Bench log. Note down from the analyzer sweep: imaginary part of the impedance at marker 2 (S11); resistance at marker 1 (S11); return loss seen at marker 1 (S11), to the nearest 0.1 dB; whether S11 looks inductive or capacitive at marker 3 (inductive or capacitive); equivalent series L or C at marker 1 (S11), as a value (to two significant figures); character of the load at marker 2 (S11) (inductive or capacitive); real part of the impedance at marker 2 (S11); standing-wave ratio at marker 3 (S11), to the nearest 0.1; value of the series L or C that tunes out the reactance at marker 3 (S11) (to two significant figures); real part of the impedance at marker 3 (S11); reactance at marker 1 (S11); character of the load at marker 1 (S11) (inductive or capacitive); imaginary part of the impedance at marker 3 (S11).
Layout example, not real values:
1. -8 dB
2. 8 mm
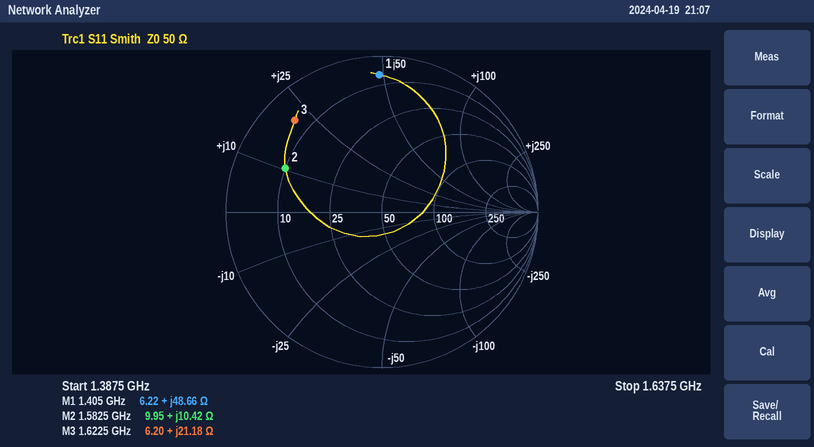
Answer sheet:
1. +10.42 Ω
2. 6.22 Ω
3. 1.1 dB
4. inductive
5. 5.5 nH
6. inductive
7. 9.95 Ω
8. 9.5
9. 4.6 pF
10. 6.20 Ω
11. +48.66 Ω
12. inductive
13. +21.18 Ω
